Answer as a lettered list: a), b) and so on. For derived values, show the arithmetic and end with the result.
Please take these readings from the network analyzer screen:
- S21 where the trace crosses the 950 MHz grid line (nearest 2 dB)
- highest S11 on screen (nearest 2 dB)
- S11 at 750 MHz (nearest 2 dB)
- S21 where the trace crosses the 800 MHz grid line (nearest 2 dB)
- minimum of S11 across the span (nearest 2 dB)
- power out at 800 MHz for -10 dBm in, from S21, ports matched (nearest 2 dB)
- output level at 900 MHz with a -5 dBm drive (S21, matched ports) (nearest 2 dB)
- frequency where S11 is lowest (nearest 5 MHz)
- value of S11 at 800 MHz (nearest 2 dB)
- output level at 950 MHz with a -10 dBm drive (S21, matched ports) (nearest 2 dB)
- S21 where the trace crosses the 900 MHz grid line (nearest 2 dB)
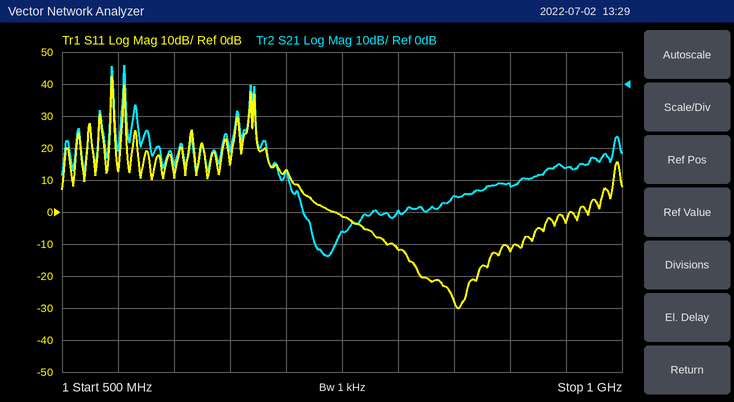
a) -26 dB
b) 42 dB
c) -2 dB
d) -40 dB
e) -30 dB
f) -10 dBm + (-40 dB) = -50 dBm
g) -5 dBm + (-32 dB) = -36 dBm
h) 855 MHz
i) -12 dB
j) -10 dBm + (-26 dB) = -36 dBm
k) -32 dB
